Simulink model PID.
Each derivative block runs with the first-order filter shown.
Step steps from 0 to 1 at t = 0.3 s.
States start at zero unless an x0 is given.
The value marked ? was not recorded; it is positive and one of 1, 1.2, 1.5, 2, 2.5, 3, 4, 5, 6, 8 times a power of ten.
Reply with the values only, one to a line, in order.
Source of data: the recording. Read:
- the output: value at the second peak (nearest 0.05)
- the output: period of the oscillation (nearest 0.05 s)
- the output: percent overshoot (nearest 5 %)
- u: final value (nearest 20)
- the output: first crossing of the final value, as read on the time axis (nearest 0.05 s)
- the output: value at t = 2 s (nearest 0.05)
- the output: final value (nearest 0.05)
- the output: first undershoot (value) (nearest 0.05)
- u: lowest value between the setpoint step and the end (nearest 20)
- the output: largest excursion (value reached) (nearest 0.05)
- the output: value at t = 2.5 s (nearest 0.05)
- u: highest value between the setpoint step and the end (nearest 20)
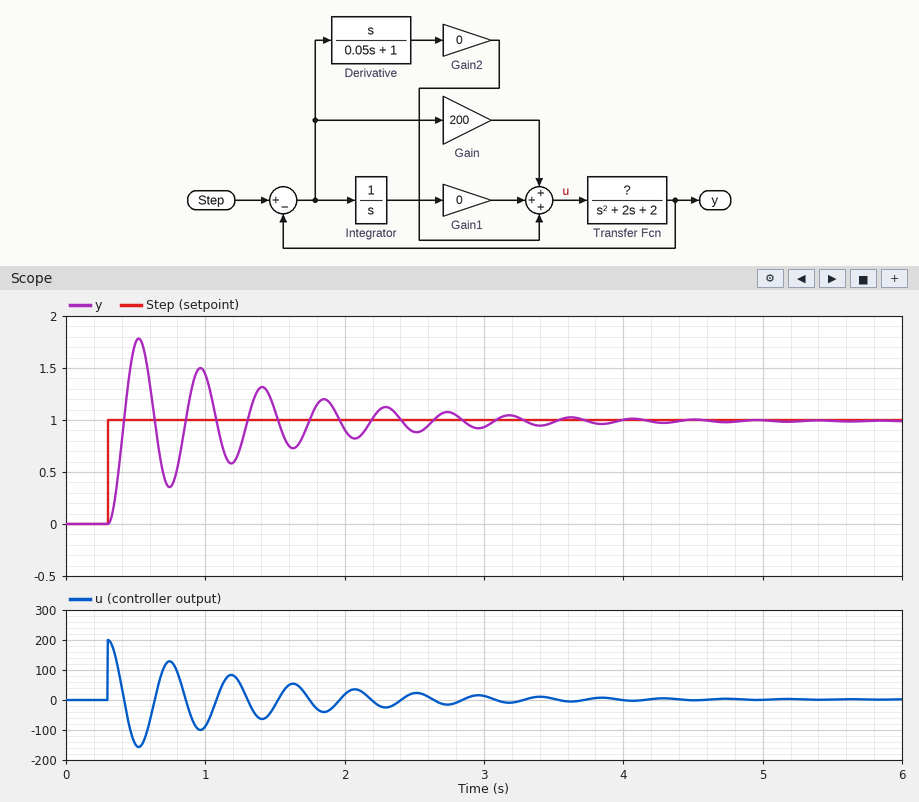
1.50
0.45 s
80 %
0
0.40 s
0.90
1.00
0.35
-160
1.80
0.90
200
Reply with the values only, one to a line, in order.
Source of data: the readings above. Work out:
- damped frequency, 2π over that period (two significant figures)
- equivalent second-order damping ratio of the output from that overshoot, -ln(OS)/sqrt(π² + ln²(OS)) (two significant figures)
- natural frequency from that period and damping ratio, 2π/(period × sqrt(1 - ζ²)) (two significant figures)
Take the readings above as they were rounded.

14 rad/s
0.071
14 rad/s
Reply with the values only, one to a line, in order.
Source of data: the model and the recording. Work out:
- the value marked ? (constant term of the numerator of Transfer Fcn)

1
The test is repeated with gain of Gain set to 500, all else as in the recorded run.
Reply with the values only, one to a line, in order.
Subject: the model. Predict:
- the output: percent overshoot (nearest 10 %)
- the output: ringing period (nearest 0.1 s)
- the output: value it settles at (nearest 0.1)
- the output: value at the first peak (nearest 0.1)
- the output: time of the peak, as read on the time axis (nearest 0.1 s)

90 %
0.3 s
1.0
1.9
0.4 s
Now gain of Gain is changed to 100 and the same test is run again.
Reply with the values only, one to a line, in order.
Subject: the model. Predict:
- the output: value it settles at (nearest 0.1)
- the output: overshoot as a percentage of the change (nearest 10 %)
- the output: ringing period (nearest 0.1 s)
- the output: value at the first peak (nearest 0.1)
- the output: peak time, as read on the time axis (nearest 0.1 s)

1.0
70 %
0.6 s
1.7
0.6 s
